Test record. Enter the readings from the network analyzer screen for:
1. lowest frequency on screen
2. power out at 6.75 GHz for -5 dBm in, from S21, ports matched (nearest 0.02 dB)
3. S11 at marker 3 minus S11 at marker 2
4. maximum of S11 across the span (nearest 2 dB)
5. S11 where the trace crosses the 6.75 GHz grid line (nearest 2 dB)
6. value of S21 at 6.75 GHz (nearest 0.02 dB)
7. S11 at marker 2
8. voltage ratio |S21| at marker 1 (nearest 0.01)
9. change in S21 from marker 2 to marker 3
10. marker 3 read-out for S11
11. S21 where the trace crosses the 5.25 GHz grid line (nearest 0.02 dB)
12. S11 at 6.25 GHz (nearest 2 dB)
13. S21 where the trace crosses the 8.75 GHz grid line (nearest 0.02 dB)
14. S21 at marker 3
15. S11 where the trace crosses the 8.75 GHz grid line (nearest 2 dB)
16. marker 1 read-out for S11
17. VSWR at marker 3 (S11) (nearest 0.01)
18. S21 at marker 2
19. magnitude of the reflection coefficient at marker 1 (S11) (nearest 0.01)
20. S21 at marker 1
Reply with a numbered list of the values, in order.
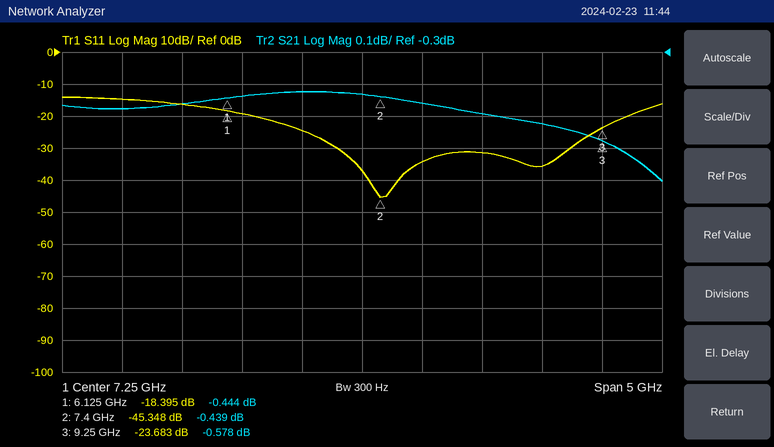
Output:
1. 4.75 GHz
2. -5.42 dBm
3. 21.665 dB
4. -14 dB
5. -24 dB
6. -0.42 dB
7. -45.348 dB
8. 0.95
9. -0.139 dB
10. -23.683 dB
11. -0.48 dB
12. -20 dB
13. -0.52 dB
14. -0.578 dB
15. -36 dB
16. -18.395 dB
17. 1.14
18. -0.439 dB
19. 0.12
20. -0.444 dB
